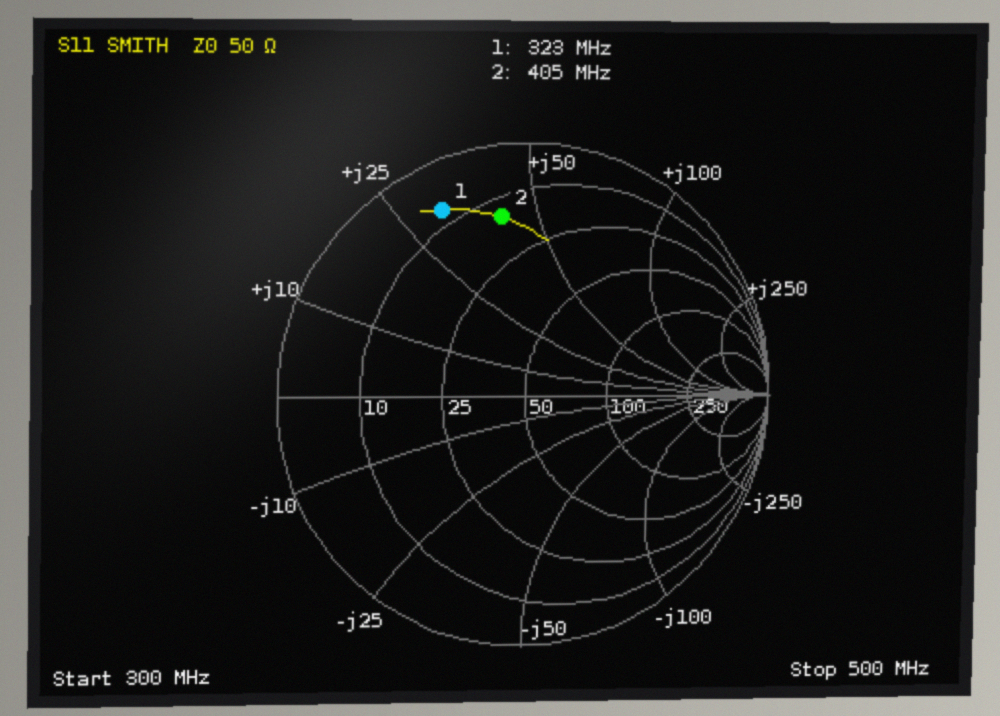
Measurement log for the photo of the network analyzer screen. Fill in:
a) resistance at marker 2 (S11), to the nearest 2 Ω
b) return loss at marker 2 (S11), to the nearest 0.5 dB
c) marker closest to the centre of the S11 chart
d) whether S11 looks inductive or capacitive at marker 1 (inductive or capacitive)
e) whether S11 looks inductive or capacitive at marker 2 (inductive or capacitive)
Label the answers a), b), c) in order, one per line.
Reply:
a) 14 Ω
b) 3.0 dB
c) marker 2
d) inductive
e) inductive
